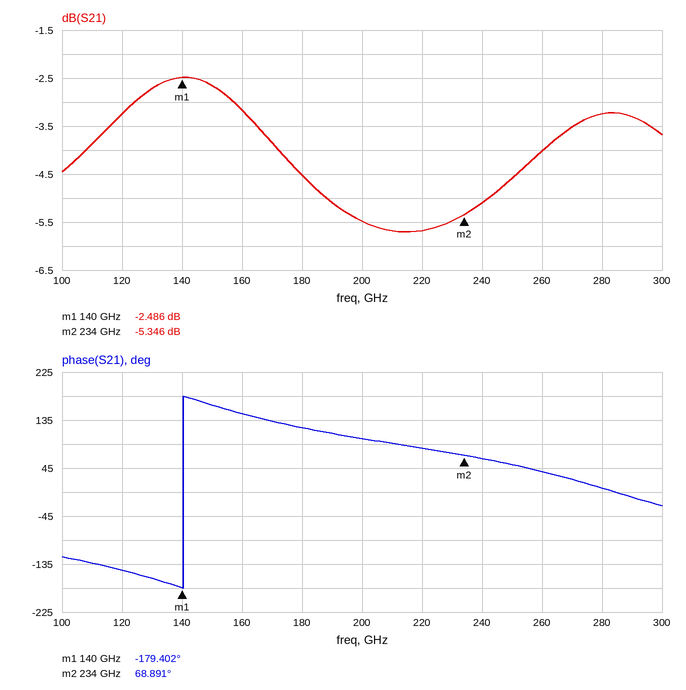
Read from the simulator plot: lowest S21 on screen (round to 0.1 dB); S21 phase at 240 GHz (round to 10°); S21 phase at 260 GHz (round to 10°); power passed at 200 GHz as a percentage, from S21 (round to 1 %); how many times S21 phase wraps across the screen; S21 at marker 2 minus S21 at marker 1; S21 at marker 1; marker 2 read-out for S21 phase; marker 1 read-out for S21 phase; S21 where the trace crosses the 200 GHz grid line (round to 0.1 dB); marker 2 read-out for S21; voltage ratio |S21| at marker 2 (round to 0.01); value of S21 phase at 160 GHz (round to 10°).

-5.7 dB
60°
40°
28 %
1
-2.860 dB
-2.486 dB
68.891°
-179.402°
-5.5 dB
-5.346 dB
0.54
150°
